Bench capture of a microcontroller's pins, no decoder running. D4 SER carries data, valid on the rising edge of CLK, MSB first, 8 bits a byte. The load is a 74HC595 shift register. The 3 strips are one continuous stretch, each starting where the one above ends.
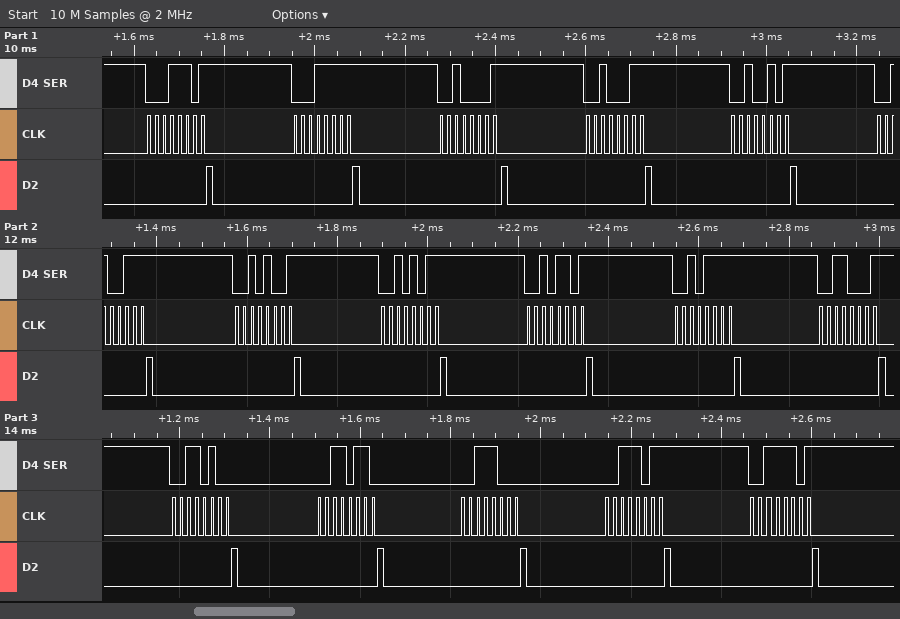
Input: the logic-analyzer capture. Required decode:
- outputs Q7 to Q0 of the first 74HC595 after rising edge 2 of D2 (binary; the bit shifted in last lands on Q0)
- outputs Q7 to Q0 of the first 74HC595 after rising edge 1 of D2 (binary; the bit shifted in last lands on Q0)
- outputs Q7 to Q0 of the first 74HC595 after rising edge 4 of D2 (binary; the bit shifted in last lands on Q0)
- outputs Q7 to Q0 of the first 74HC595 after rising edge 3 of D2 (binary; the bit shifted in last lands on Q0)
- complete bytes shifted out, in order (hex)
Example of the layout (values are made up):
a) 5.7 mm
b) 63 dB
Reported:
a) 00011111
b) 00011101
c) 00100011
d) 00100001
e) 0x1D 0x1F 0x21 0x23 0x25 0x27 0x29 0x2B 0x2D 0x2F 0x31 0x34 0x36 0x38 0x3B 0x3D
